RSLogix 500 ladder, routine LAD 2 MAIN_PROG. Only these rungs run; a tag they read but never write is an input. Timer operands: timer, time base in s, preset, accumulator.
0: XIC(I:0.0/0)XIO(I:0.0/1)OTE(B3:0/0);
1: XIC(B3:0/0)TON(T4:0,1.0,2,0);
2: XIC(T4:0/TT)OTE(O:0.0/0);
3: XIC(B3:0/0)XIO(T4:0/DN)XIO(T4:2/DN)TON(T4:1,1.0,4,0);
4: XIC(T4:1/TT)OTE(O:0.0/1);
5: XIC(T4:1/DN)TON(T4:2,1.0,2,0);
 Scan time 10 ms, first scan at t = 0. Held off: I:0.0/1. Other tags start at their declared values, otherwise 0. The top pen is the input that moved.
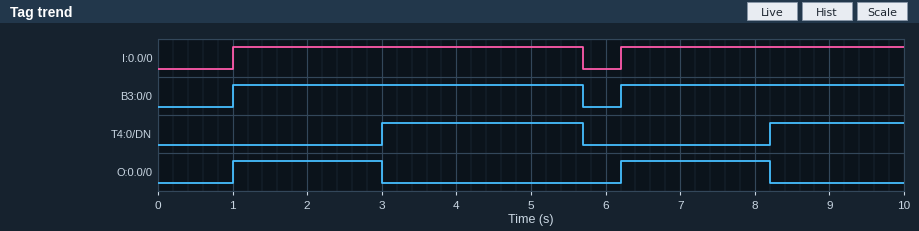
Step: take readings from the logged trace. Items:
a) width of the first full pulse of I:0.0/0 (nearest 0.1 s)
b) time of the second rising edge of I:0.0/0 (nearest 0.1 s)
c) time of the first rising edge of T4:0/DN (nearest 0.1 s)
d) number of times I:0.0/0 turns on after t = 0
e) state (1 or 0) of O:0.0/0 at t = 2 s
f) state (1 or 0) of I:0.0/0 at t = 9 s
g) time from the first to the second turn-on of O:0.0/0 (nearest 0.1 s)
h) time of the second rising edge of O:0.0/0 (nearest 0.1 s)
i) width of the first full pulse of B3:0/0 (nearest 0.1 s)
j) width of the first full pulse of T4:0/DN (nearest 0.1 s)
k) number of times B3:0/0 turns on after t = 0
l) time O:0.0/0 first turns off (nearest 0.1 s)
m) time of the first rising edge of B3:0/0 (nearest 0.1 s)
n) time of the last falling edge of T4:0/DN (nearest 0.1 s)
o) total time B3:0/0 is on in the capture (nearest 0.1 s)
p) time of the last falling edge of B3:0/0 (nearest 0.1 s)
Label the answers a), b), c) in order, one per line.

a) 4.7 s
b) 6.2 s
c) 3.0 s
d) 2
e) 1
f) 1
g) 5.2 s
h) 6.2 s
i) 4.7 s
j) 2.7 s
k) 2
l) 3.0 s
m) 1.0 s
n) 5.7 s
o) 8.5 s
p) 5.7 s
